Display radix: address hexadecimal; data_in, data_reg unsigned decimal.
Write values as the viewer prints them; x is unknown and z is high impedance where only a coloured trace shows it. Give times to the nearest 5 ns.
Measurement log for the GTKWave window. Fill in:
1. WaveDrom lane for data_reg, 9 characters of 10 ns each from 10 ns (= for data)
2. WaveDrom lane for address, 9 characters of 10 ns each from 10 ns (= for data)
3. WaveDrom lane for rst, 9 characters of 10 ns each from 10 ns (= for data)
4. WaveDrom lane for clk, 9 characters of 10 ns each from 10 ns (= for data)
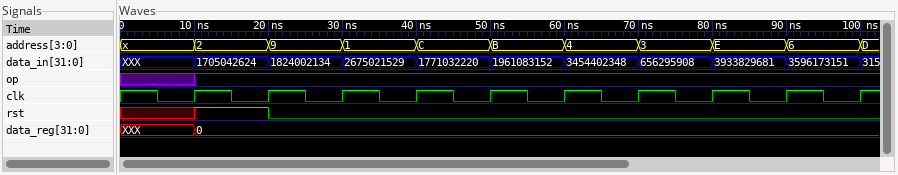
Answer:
{name: 'data_reg', wave: '=........', data: '0'}
{name: 'address', wave: '=========', data: '2 9 1 C B 4 3 E 6'}
{name: 'rst', wave: '10.......'}
{name: 'clk', wave: 'p........'}
